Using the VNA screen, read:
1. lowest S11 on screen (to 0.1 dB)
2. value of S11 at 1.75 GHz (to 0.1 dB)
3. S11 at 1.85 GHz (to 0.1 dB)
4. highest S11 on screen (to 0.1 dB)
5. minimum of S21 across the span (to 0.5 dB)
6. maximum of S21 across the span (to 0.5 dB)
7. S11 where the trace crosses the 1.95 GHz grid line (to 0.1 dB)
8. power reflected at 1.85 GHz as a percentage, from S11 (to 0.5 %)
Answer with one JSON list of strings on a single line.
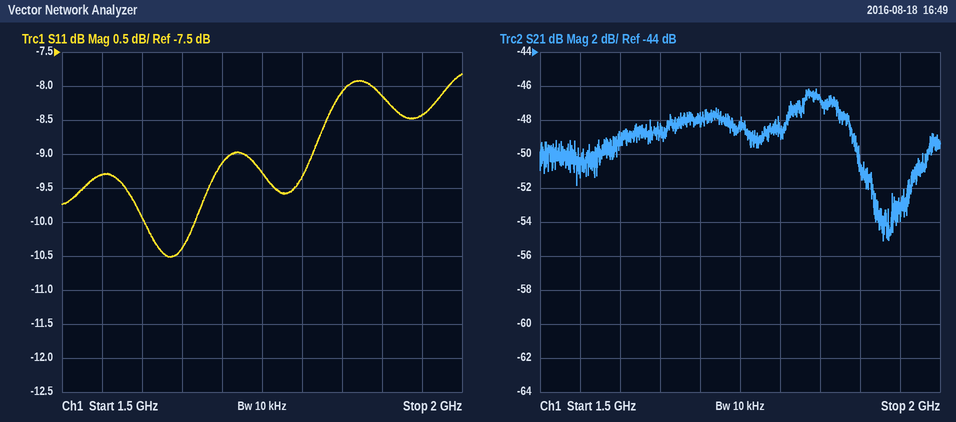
["-10.5 dB", "-9.3 dB", "-8.1 dB", "-7.8 dB", "-55.0 dB", "-46.0 dB", "-8.4 dB", "15.5 %"]
